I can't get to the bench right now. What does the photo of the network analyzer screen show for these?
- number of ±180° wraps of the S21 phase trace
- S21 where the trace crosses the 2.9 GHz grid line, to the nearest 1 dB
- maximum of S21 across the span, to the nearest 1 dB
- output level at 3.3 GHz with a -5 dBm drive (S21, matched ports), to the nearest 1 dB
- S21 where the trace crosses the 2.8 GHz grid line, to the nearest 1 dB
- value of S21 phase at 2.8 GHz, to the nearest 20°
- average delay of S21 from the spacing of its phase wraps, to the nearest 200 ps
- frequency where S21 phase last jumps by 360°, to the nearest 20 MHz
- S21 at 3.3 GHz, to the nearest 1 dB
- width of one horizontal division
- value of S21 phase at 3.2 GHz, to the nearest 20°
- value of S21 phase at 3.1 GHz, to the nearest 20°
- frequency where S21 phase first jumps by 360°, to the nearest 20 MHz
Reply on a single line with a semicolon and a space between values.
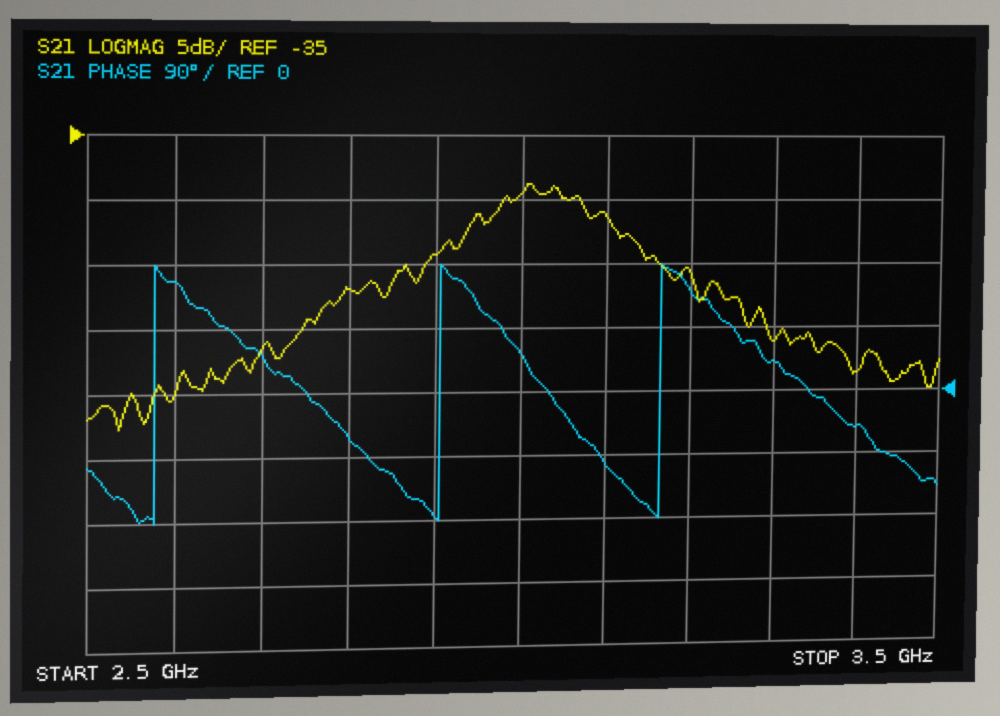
3; -44 dB; -39 dB; -56 dBm; -47 dB; -60°; 3.4 ns; 3.16 GHz; -51 dB; 100 MHz; 140°; -100°; 2.58 GHz
